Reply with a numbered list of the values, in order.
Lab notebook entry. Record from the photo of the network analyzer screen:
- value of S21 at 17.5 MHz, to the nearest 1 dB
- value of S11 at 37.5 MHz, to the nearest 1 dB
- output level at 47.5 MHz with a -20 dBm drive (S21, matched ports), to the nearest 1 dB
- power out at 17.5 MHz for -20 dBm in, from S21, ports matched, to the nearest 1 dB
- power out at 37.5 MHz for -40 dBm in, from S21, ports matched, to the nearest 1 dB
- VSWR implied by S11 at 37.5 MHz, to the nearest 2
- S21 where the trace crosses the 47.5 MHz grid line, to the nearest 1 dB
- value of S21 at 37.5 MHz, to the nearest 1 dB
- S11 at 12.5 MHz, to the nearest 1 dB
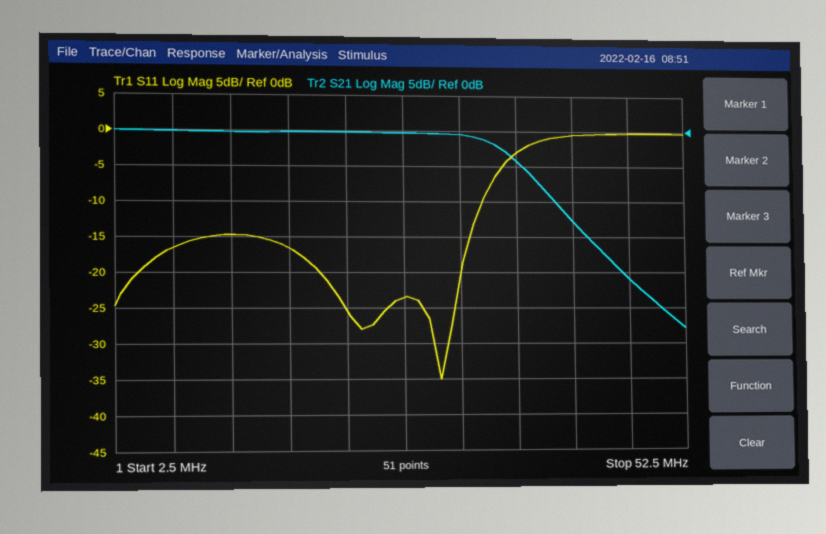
1. 0 dB
2. -3 dB
3. -41 dBm
4. -20 dBm
5. -44 dBm
6. 6
7. -21 dB
8. -4 dB
9. -15 dB
